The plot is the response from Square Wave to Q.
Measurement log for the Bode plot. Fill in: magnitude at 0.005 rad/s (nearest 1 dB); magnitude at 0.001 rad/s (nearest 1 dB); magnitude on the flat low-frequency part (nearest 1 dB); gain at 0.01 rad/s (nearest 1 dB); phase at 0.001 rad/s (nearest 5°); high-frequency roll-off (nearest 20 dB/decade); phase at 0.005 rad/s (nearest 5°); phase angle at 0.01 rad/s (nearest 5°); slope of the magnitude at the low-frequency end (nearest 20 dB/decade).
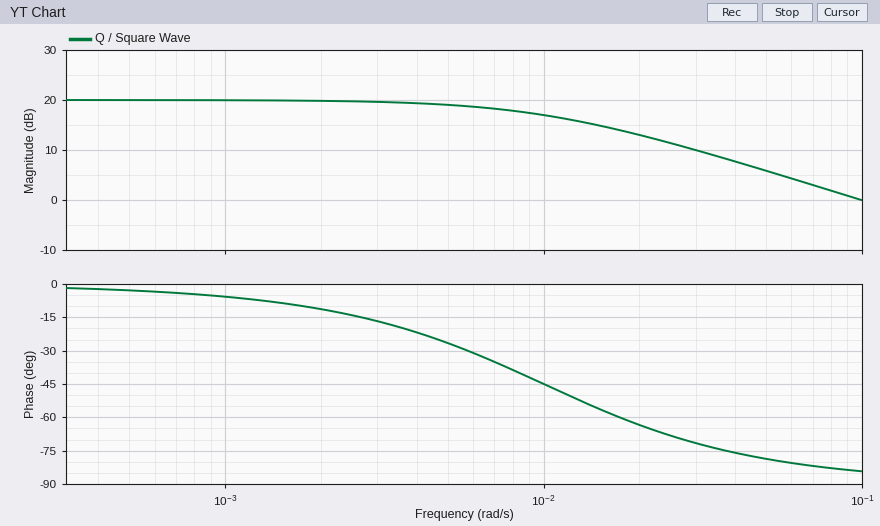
19 dB
20 dB
20 dB
17 dB
-5°
-20 dB/decade
-25°
-45°
0 dB/decade
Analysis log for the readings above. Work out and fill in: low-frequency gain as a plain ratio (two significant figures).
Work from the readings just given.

10
